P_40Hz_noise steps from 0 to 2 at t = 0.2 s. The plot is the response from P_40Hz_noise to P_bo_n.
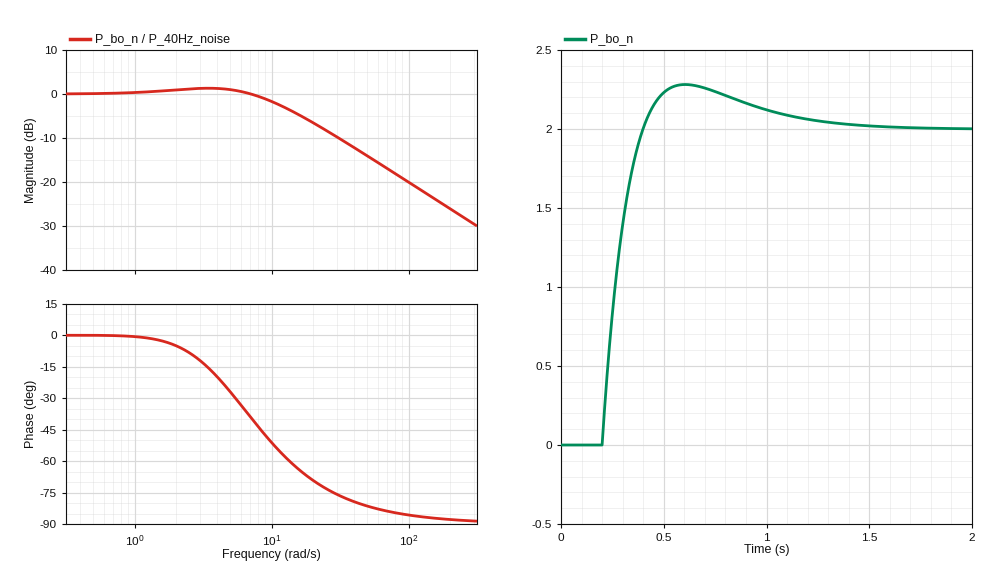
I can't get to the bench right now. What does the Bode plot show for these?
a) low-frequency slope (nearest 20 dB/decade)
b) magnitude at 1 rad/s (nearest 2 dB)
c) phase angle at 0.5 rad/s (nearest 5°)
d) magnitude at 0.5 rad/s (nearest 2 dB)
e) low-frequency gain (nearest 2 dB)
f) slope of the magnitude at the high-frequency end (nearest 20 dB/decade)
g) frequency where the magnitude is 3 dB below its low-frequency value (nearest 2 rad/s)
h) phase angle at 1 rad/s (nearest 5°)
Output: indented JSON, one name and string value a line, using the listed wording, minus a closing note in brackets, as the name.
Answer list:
{
  "low-frequency slope": "0 dB/decade",
  "magnitude at 1 rad/s": "0 dB",
  "phase angle at 0.5 rad/s": "0°",
  "magnitude at 0.5 rad/s": "0 dB",
  "low-frequency gain": "0 dB",
  "slope of the magnitude at the high-frequency end": "-20 dB/decade",
  "frequency where the magnitude is 3 dB below its low-frequency value": "12 rad/s",
  "phase angle at 1 rad/s": "0°"
}
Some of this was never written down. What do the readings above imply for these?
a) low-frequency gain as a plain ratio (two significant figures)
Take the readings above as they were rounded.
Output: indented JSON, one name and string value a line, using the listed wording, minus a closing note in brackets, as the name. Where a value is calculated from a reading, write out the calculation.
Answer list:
{
  "low-frequency gain as a plain ratio": "10^(0 / 20) = 1.0"
}
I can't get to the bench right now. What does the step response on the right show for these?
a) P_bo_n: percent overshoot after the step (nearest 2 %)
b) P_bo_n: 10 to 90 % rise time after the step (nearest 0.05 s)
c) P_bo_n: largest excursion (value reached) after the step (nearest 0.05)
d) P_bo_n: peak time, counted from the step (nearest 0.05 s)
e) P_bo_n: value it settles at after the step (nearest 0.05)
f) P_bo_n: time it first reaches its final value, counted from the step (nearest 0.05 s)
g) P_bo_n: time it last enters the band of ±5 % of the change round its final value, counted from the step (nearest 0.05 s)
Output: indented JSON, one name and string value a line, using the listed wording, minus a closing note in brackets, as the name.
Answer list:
{
  "P_bo_n: percent overshoot after the step": "14 %",
  "P_bo_n: 10 to 90 % rise time after the step": "0.15 s",
  "P_bo_n: largest excursion (value reached) after the step": "2.30",
  "P_bo_n: peak time, counted from the step": "0.40 s",
  "P_bo_n: value it settles at after the step": "2.00",
  "P_bo_n: time it first reaches its final value, counted from the step": "0.20 s",
  "P_bo_n: time it last enters the band of ±5 % of the change round its final value, counted from the step": "0.85 s"
}
